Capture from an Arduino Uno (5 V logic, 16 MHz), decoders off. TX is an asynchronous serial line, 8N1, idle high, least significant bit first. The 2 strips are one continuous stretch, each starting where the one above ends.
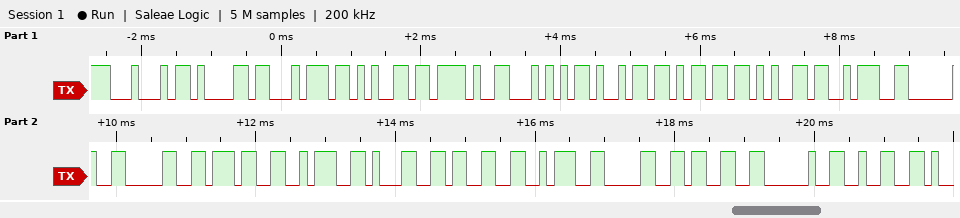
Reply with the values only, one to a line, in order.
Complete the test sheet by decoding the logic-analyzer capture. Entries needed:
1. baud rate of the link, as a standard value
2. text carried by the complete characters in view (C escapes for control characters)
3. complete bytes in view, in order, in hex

9600 baud
"Date/Time: 07:13:03 2"
44 61 74 65 2F 54 69 6D 65 3A 20 30 37 3A 31 33 3A 30 33 20 32
